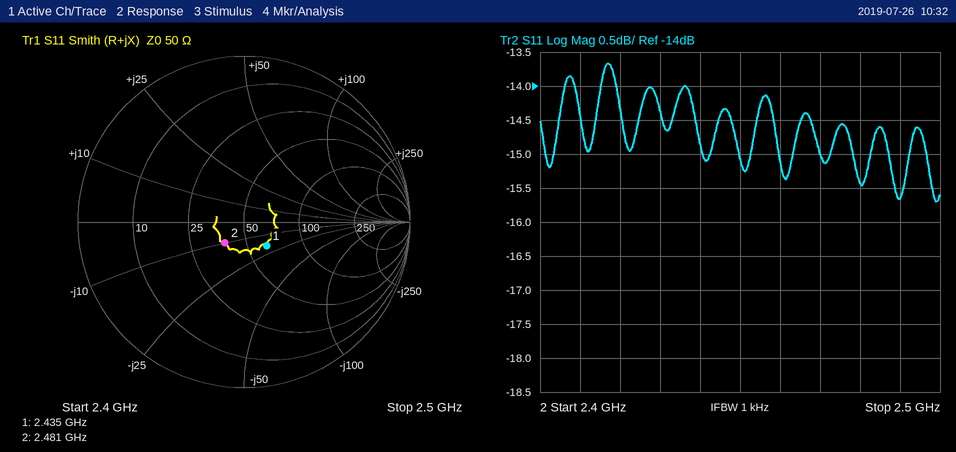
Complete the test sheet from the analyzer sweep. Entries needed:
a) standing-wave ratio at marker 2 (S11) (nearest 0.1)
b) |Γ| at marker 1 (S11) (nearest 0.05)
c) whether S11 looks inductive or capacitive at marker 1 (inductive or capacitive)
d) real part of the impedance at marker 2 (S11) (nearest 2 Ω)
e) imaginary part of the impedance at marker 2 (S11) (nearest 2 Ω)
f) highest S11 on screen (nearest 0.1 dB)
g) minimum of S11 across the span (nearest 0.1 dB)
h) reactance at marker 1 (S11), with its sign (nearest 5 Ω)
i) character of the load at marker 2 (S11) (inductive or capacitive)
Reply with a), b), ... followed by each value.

a) 1.4
b) 0.20
c) capacitive
d) 38 Ω
e) -10 Ω
f) -13.7 dB
g) -15.7 dB
h) -20 Ω
i) capacitive
